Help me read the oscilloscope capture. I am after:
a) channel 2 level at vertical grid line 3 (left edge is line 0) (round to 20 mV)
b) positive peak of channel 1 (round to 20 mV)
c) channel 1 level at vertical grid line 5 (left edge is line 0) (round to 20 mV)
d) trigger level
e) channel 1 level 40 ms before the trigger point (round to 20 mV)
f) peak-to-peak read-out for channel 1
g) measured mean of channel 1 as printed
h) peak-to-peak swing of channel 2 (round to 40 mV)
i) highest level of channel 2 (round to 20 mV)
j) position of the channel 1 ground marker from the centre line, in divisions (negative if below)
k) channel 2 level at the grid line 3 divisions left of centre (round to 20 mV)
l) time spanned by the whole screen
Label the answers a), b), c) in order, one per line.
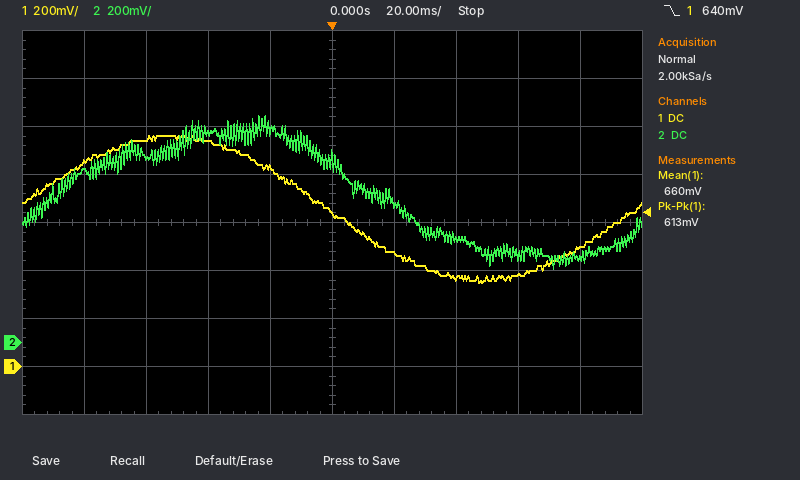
a) 880 mV
b) 960 mV
c) 640 mV
d) 640 mV
e) 940 mV
f) 613 mV
g) 660 mV
h) 640 mV
i) 940 mV
j) -3.0 div
k) 780 mV
l) 200 ms
